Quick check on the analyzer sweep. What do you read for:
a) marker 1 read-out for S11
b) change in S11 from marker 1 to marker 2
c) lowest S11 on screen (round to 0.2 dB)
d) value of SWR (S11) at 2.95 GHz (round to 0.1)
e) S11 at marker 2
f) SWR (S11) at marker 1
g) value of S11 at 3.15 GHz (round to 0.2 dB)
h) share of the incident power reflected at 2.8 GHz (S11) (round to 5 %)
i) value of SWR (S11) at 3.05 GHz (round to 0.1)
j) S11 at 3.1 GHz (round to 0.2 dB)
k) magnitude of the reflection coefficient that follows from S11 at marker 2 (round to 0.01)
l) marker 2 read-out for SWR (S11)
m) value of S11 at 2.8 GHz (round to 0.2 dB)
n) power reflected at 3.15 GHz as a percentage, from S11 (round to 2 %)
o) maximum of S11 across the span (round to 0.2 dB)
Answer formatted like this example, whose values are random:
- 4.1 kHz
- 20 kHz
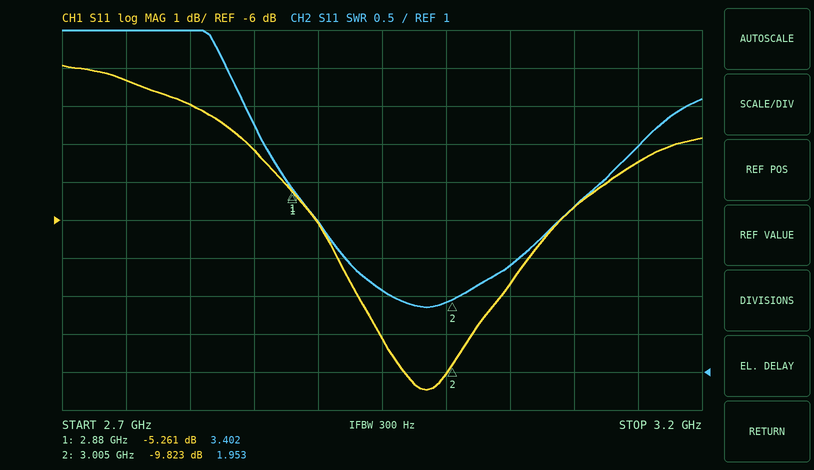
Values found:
- -5.261 dB
- -4.562 dB
- -10.4 dB
- 2.1
- -9.823 dB
- 3.402
- -4.4 dB
- 50 %
- 2.4
- -5.6 dB
- 0.32
- 1.953
- -3.0 dB
- 36 %
- -2.0 dB
